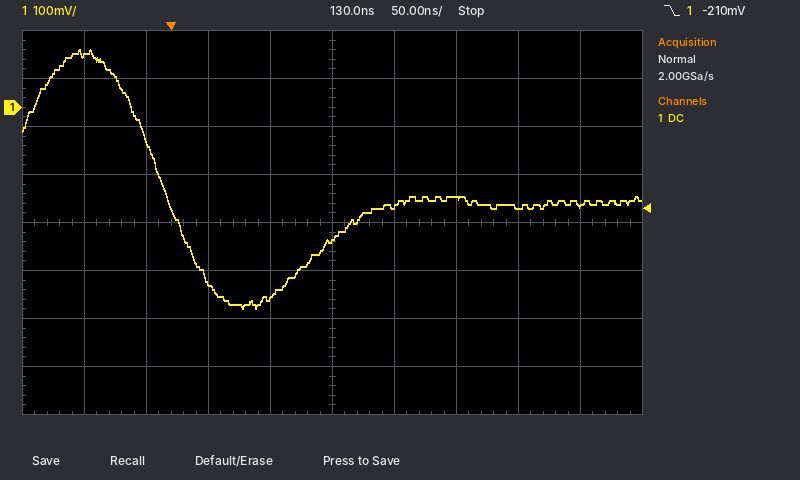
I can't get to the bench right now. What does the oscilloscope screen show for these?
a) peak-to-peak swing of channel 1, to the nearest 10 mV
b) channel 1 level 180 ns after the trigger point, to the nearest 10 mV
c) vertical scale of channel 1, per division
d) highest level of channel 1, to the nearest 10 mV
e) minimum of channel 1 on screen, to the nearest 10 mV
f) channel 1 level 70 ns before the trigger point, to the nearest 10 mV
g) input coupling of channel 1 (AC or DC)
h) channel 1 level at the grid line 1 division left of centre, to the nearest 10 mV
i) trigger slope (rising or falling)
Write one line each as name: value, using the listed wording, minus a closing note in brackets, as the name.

peak-to-peak swing of channel 1, to the nearest 10 mV: 540 mV
channel 1 level 180 ns after the trigger point, to the nearest 10 mV: -210 mV
vertical scale of channel 1, per division: 100 mV
highest level of channel 1, to the nearest 10 mV: 120 mV
minimum of channel 1 on screen, to the nearest 10 mV: -420 mV
channel 1 level 70 ns before the trigger point, to the nearest 10 mV: 110 mV
input coupling of channel 1: DC
channel 1 level at the grid line 1 division left of centre, to the nearest 10 mV: -400 mV
trigger slope: falling
